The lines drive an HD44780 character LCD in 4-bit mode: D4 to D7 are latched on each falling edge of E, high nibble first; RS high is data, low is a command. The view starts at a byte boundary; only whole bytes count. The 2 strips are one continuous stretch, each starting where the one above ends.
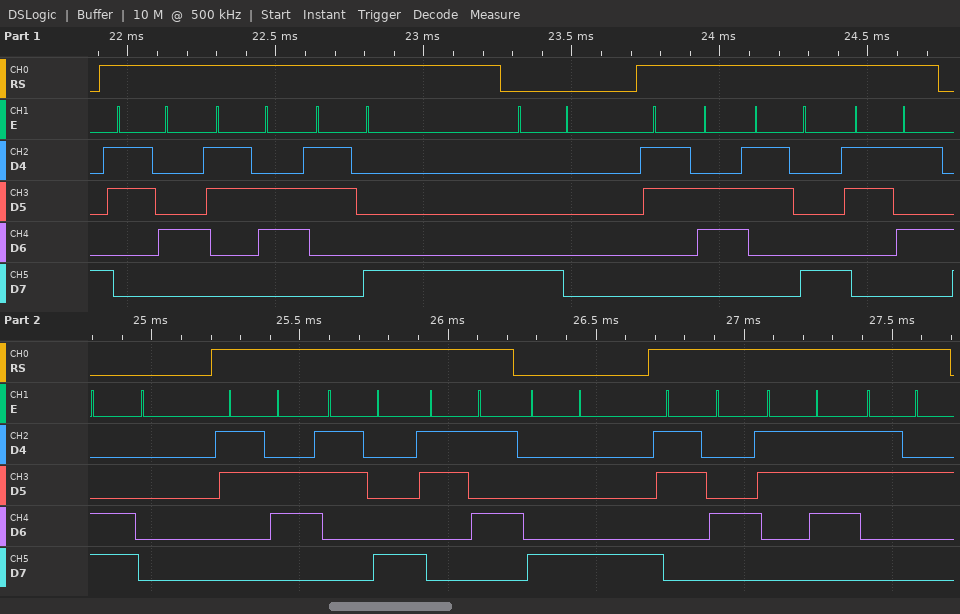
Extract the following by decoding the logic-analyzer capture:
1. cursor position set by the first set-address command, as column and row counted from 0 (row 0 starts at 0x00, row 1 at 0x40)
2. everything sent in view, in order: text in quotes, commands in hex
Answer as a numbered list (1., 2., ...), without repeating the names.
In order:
1. column 0, row 0
2. "468" 0x80 "685" 0xC0 "685" 0x88 "472"
